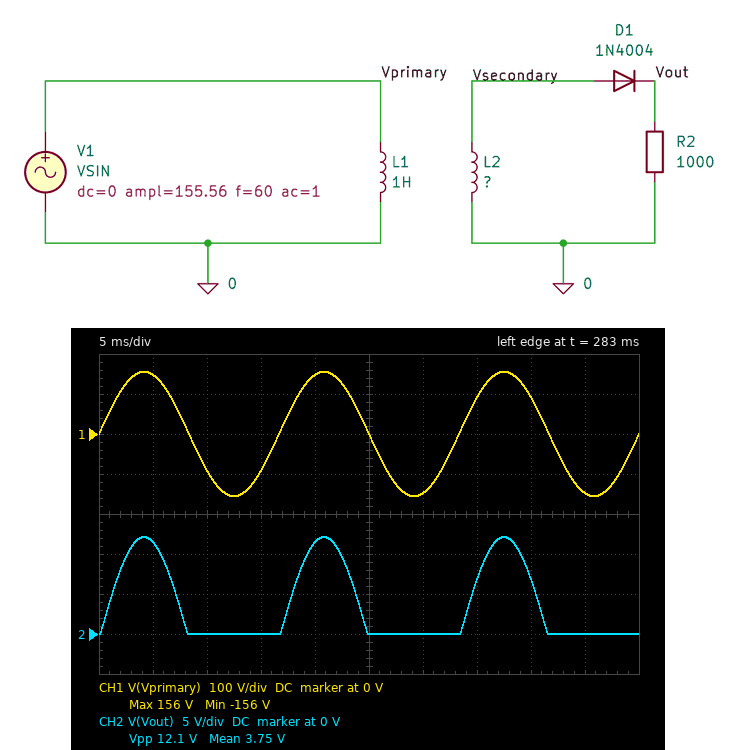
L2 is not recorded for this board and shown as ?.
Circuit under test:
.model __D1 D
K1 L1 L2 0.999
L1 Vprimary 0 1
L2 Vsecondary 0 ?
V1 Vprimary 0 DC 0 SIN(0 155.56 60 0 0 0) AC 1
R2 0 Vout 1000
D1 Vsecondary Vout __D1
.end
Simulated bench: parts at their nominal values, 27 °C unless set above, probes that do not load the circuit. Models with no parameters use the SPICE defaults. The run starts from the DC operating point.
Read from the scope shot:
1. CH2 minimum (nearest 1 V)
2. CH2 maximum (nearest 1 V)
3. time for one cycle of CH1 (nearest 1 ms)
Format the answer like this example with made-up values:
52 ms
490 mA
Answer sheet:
0 V
12 V
17 ms
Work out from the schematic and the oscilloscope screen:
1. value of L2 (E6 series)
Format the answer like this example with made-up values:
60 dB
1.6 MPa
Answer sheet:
6.8 mH
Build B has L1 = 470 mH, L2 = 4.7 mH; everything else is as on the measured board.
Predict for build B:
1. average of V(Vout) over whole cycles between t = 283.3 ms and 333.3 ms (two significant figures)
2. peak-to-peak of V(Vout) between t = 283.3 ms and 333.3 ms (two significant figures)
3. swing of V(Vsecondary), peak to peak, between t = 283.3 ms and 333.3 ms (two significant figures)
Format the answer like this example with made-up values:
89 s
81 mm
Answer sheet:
4.6 V
15 V
31 V
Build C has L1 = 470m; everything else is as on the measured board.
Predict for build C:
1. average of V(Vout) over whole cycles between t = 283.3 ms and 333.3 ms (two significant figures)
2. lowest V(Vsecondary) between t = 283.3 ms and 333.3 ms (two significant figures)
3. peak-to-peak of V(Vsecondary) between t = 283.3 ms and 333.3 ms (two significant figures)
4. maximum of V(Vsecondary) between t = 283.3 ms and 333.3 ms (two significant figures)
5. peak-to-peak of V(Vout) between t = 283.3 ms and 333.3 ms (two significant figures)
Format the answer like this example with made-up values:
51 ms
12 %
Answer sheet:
5.6 V
-19 V
37 V
19 V
18 V
